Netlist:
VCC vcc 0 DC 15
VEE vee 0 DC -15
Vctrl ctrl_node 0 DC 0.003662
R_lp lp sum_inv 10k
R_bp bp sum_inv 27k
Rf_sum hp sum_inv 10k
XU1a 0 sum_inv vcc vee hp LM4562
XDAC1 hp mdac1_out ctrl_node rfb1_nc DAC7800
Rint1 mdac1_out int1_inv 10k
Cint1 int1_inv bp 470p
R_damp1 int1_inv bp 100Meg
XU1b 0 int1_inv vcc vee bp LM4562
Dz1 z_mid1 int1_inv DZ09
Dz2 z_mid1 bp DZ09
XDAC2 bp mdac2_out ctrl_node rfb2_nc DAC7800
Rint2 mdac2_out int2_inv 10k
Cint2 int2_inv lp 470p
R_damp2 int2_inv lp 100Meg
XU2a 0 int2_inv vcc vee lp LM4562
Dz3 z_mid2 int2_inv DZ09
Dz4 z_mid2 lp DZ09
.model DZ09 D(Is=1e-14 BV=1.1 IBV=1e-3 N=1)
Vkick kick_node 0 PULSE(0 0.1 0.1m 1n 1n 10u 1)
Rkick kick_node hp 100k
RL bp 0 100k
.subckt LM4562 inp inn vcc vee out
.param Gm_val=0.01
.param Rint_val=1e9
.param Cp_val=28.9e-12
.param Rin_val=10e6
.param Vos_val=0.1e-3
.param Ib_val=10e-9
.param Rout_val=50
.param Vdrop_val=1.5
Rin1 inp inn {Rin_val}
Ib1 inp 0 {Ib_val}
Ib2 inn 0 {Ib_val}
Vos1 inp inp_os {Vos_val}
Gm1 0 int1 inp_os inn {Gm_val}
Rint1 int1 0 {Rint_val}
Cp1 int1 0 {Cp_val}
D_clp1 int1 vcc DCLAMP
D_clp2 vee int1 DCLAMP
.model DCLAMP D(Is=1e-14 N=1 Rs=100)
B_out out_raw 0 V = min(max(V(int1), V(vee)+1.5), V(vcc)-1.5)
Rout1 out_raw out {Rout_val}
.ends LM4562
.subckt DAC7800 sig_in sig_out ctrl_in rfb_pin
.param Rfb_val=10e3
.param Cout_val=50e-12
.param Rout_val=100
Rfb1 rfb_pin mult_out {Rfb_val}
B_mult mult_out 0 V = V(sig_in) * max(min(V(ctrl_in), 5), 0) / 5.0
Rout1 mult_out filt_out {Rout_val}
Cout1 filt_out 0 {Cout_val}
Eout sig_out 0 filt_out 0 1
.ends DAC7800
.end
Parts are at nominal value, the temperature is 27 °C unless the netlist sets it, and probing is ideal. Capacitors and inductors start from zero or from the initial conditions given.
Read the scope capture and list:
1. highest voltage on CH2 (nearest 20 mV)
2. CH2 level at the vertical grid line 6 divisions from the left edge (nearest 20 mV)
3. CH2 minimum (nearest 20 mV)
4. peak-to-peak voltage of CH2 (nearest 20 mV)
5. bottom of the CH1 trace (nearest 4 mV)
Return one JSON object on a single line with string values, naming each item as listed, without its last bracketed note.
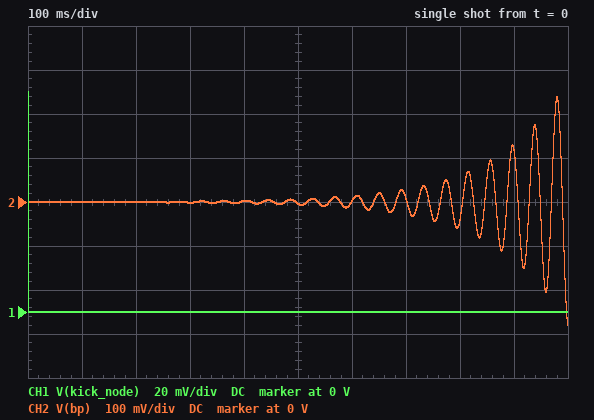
{"highest voltage on CH2": "240 mV", "CH2 level at the vertical grid line 6 divisions from the left edge": "0 V", "CH2 minimum": "-280 mV", "peak-to-peak voltage of CH2": "520 mV", "bottom of the CH1 trace": "0 V"}
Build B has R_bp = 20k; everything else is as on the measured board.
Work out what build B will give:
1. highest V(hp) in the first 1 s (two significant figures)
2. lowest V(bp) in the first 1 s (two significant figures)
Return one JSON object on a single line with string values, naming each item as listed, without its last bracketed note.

{"highest V(hp) in the first 1 s": "1.2 V", "lowest V(bp) in the first 1 s": "-1.2 V"}
